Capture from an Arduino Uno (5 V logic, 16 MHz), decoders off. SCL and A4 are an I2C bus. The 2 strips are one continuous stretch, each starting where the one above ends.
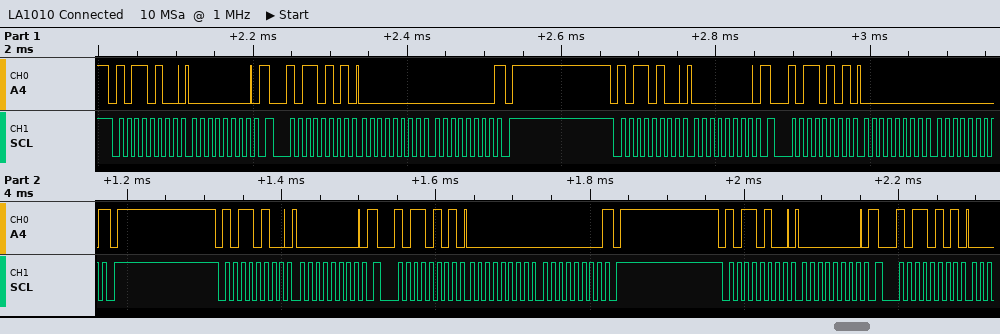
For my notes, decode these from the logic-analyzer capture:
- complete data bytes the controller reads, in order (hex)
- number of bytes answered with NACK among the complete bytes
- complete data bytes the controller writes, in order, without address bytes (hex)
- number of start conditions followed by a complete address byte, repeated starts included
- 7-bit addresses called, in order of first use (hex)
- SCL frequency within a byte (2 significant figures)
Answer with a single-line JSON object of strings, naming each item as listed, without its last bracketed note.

{"complete data bytes the controller reads, in order": "00 00 00 00 00 00", "number of bytes answered with NACK among the complete bytes": "3", "complete data bytes the controller writes, in order, without address bytes": "00 00 00 00", "number of start conditions followed by a complete address byte, repeated starts included": "8", "7-bit addresses called, in order of first use": "0x5A", "SCL frequency within a byte": "100 kHz"}
